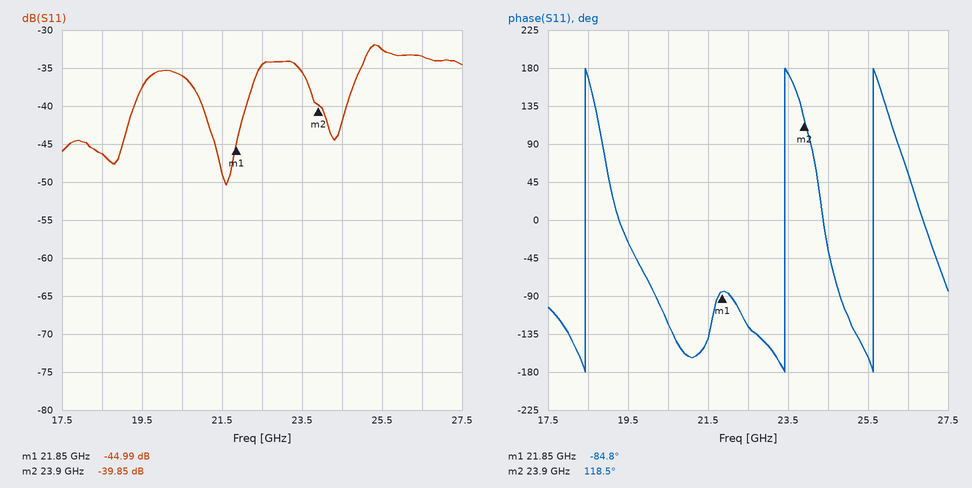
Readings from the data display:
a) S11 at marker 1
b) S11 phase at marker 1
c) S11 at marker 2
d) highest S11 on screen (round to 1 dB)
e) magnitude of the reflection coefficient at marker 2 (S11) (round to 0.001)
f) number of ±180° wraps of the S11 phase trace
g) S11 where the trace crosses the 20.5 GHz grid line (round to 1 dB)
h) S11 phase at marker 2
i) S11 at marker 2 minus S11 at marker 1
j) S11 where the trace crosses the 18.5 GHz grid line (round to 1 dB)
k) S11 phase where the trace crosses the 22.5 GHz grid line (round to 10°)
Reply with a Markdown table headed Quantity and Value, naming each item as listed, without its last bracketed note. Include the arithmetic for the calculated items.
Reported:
| Quantity | Value |
|---|---|
| S11 at marker 1 | -44.99 dB |
| S11 phase at marker 1 | -84.8° |
| S11 at marker 2 | -39.85 dB |
| highest S11 on screen | -32 dB |
| magnitude of the reflection coefficient at marker 2 (S11) | 10^(-39.85/20) ≈ 0.010 |
| number of ±180° wraps of the S11 phase trace | 3 |
| S11 where the trace crosses the 20.5 GHz grid line | -36 dB |
| S11 phase at marker 2 | 118.5° |
| S11 at marker 2 minus S11 at marker 1 | -39.85 − (-44.99) = 5.14 dB |
| S11 where the trace crosses the 18.5 GHz grid line | -46 dB |
| S11 phase where the trace crosses the 22.5 GHz grid line | -130° |
